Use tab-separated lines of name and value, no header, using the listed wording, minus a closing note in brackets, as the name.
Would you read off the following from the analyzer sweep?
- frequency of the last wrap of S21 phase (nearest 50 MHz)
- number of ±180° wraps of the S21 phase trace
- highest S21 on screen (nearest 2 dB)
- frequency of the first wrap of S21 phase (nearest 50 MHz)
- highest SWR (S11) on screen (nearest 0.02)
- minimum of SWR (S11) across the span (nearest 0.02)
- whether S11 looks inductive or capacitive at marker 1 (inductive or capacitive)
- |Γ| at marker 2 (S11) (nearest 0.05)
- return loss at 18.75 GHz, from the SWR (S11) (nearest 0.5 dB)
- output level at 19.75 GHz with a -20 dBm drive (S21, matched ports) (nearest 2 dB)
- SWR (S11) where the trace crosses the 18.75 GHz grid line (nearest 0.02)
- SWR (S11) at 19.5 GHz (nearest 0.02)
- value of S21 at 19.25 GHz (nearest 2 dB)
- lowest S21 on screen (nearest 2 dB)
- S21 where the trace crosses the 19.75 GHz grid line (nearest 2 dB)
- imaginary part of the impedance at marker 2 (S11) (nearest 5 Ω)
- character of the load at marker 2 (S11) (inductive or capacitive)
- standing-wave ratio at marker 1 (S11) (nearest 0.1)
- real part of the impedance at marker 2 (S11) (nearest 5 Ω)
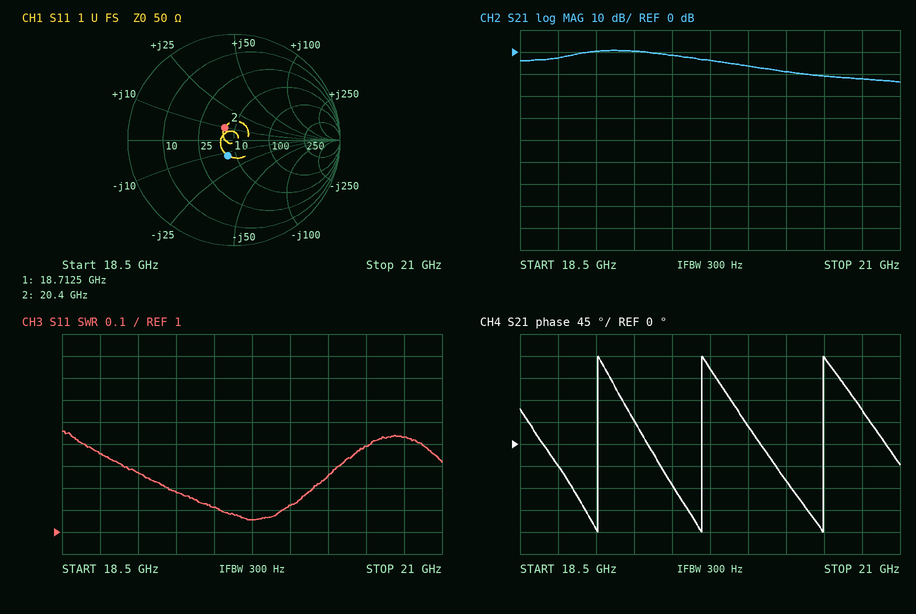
frequency of the last wrap of S21 phase	20.50 GHz
number of ±180° wraps of the S21 phase trace	3
highest S21 on screen	0 dB
frequency of the first wrap of S21 phase	19.00 GHz
highest SWR (S11) on screen	1.46
minimum of SWR (S11) across the span	1.06
whether S11 looks inductive or capacitive at marker 1	capacitive
|Γ| at marker 2 (S11)	0.15
return loss at 18.75 GHz, from the SWR (S11)	16.5 dB
output level at 19.75 GHz with a -20 dBm drive (S21, matched ports)	-24 dBm
SWR (S11) where the trace crosses the 18.75 GHz grid line	1.36
SWR (S11) at 19.5 GHz	1.12
value of S21 at 19.25 GHz	0 dB
lowest S21 on screen	-14 dB
S21 where the trace crosses the 19.75 GHz grid line	-4 dB
imaginary part of the impedance at marker 2 (S11)	+10 Ω
character of the load at marker 2 (S11)	inductive
standing-wave ratio at marker 1 (S11)	1.4
real part of the impedance at marker 2 (S11)	40 Ω
